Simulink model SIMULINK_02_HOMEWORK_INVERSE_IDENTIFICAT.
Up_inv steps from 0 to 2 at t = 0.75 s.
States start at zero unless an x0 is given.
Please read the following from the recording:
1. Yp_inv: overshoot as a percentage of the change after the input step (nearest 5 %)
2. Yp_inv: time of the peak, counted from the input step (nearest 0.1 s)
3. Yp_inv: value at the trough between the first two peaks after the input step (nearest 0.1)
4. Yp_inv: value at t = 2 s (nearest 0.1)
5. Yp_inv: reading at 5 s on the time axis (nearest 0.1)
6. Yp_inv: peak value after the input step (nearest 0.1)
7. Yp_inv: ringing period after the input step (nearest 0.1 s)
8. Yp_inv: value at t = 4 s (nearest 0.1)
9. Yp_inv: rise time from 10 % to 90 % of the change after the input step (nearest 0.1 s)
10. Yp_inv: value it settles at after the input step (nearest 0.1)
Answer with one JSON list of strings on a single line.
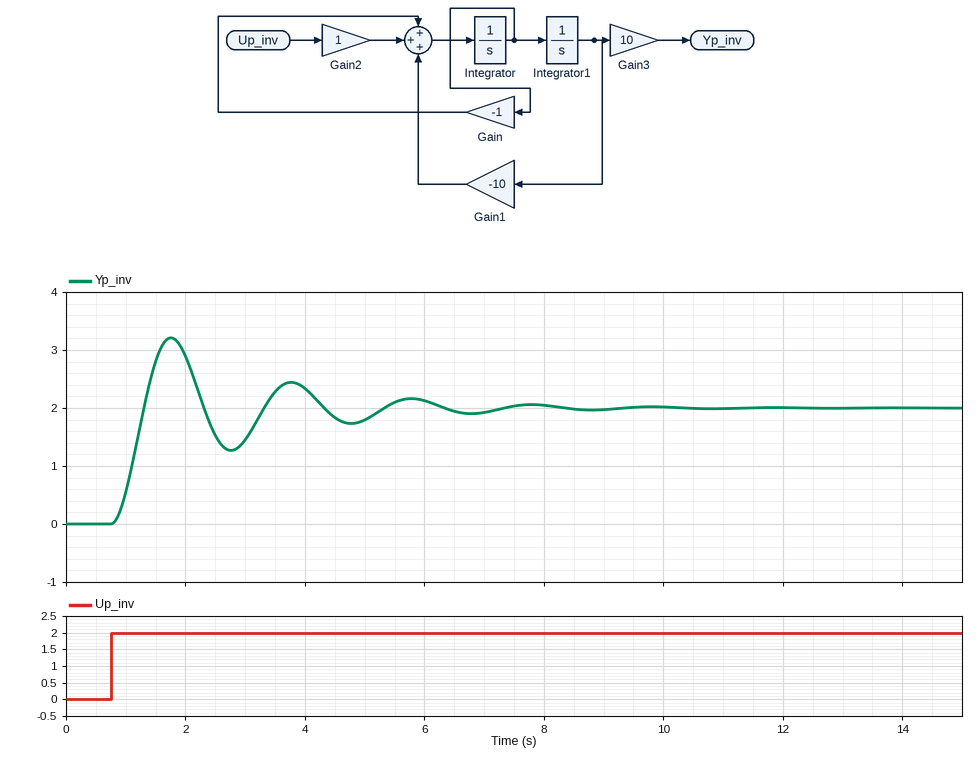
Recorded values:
["60 %", "1.0 s", "1.3", "2.9", "1.8", "3.2", "2.0 s", "2.3", "0.4 s", "2.0"]
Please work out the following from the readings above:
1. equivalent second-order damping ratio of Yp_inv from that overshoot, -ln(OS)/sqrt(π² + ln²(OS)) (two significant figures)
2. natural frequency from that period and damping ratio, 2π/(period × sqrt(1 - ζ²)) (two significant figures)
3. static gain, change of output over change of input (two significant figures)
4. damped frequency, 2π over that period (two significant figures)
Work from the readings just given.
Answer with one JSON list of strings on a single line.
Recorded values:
["0.16", "3.2 rad/s", "1.0", "3.1 rad/s"]
